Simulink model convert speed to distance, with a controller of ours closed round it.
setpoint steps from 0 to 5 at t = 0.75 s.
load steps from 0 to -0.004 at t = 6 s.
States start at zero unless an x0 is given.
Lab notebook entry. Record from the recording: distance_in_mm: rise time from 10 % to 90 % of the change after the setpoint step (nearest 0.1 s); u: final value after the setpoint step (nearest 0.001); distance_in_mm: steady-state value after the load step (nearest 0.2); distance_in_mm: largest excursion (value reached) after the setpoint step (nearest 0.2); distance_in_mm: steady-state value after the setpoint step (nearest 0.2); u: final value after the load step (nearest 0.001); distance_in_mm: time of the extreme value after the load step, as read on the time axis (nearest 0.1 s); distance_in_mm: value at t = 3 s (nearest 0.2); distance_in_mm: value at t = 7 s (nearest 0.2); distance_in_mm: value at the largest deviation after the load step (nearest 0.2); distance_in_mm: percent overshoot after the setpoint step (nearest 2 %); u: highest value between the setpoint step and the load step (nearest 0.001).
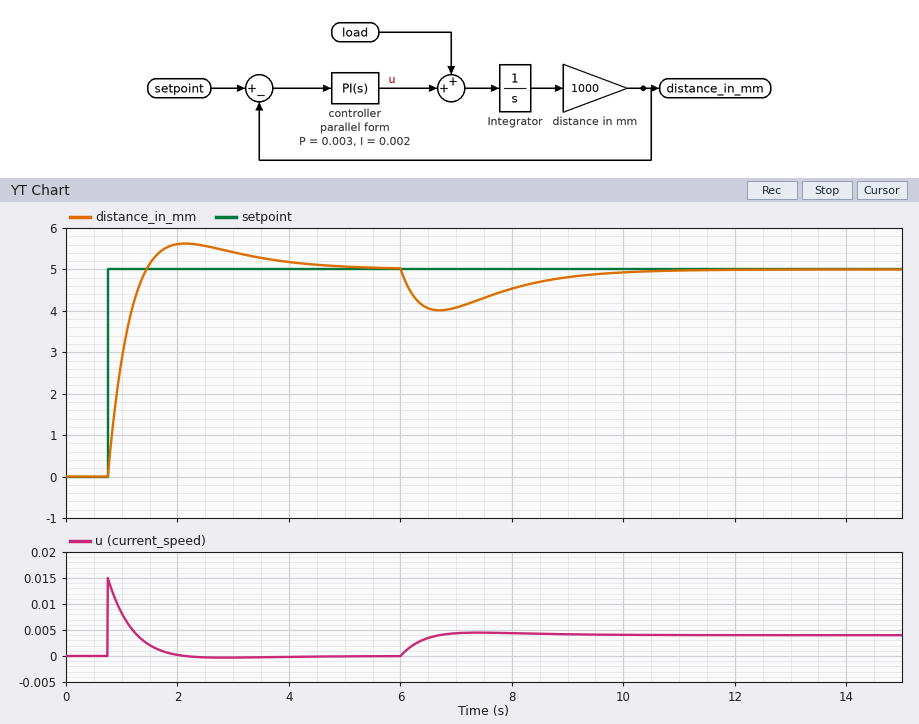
0.5 s
0.000
5.0
5.6
5.0
0.004
6.7 s
5.4
4.0
4.0
12 %
0.015
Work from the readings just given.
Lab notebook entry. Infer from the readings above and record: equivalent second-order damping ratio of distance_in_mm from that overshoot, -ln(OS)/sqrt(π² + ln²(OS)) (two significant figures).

0.56
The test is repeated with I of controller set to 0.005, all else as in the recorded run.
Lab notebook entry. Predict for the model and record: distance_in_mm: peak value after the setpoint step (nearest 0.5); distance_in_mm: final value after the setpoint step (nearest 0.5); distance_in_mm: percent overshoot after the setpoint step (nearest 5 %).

6.0
5.0
20 %
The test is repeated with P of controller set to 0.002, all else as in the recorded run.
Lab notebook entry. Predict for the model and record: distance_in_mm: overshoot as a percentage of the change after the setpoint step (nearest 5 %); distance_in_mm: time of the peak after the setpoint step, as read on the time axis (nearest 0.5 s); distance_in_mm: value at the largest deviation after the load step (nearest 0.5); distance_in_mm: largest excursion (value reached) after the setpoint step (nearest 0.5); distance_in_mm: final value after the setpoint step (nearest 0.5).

20 %
2.5 s
3.5
6.0
5.0
